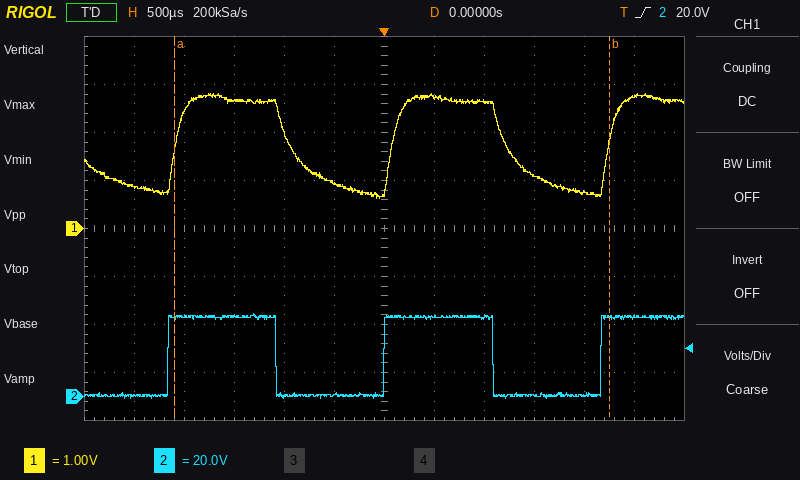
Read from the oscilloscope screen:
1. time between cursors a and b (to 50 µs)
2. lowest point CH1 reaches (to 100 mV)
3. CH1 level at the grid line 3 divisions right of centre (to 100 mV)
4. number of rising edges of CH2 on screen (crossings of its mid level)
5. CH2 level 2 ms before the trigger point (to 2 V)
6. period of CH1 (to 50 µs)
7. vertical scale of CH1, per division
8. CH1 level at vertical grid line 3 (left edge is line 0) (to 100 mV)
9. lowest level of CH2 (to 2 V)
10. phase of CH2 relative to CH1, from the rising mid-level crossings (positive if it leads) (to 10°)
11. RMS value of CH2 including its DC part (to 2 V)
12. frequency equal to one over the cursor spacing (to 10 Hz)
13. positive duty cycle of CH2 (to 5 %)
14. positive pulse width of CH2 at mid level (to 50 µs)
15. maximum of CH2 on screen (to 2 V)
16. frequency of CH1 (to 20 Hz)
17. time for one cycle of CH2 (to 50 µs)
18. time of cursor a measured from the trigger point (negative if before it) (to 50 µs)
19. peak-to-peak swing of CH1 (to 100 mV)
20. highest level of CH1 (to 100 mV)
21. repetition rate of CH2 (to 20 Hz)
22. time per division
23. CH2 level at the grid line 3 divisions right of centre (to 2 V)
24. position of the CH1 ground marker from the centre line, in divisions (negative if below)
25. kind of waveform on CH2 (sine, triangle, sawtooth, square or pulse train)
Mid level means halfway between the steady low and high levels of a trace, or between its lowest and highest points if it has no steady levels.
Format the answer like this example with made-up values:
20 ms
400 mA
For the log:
4.35 ms
600 mV
1.1 V
3
34 V
2.15 ms
1 V
2.7 V
0 V
+10°
24 V
230 Hz
50 %
1.10 ms
34 V
460 Hz
2.15 ms
-2.10 ms
2.2 V
2.8 V
460 Hz
500 µs
0 V
0.0 div
square
